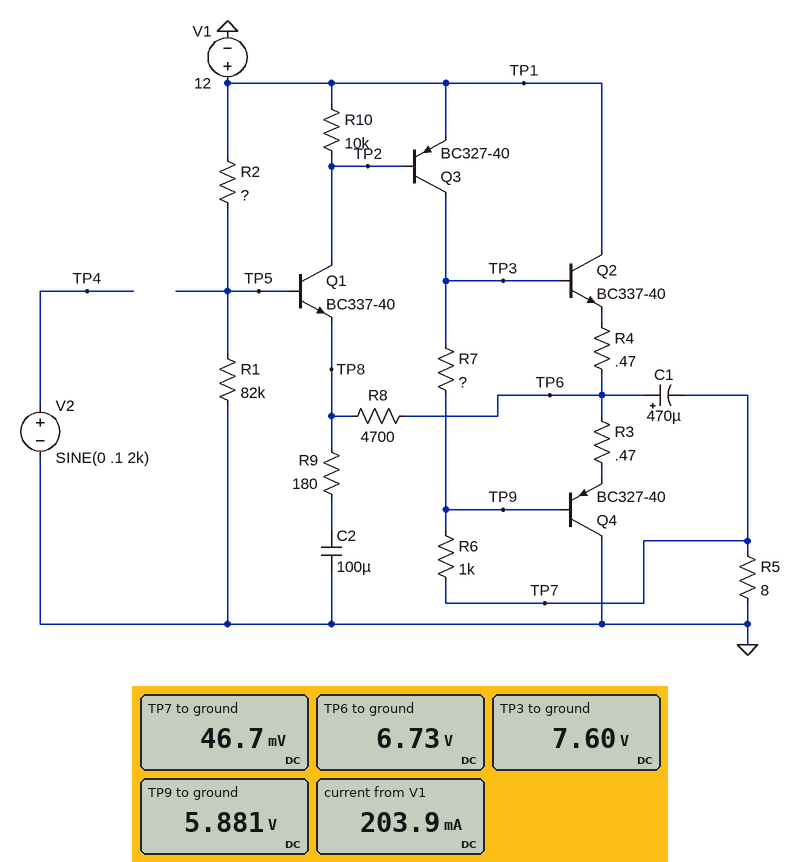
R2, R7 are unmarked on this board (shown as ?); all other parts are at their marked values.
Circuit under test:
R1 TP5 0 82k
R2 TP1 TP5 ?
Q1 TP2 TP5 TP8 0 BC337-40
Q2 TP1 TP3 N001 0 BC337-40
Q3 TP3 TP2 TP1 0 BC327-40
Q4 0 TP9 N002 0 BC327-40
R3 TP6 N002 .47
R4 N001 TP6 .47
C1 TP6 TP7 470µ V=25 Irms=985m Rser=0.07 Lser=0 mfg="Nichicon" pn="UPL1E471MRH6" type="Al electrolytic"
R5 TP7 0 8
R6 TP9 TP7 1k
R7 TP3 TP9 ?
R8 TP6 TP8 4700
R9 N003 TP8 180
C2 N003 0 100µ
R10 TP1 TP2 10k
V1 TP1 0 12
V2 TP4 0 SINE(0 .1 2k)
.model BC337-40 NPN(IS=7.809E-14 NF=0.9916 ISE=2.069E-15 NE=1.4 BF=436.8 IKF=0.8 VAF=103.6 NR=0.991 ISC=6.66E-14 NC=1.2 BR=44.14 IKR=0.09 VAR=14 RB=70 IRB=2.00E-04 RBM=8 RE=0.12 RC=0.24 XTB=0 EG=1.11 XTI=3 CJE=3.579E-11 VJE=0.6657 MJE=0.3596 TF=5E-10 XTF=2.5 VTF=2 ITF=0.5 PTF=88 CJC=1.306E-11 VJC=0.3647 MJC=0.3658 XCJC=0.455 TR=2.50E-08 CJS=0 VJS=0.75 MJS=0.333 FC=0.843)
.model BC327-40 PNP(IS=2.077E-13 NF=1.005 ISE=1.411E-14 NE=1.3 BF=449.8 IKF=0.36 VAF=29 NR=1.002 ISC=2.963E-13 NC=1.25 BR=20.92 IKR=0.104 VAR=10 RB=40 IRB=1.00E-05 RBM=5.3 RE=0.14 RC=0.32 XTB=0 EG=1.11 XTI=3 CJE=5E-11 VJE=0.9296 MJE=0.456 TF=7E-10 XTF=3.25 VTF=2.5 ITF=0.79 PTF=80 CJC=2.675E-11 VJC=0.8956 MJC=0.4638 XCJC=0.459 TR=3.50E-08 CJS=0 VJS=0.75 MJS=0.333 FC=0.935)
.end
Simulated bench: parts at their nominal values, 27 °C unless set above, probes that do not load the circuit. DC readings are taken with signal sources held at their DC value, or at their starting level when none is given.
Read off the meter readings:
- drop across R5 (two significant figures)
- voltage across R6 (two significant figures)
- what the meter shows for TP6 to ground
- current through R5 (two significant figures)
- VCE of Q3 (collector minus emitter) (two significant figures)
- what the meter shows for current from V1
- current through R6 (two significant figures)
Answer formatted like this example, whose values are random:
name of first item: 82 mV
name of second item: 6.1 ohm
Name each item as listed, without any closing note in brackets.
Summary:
drop across R5: 47 mV
voltage across R6: 5.8 V
what the meter shows for TP6 to ground: 6.73 V
current through R5: 5.8 mA
VCE of Q3 (collector minus emitter): -4.4 V
what the meter shows for current from V1: 203.9 mA
current through R6: 5.8 mA
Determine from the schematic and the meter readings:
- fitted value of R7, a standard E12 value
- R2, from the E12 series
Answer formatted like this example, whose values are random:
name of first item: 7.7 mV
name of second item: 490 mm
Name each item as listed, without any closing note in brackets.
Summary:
fitted value of R7, a standard E12 value: 330 Ω
R2, from the E12 series: 47 kΩ
